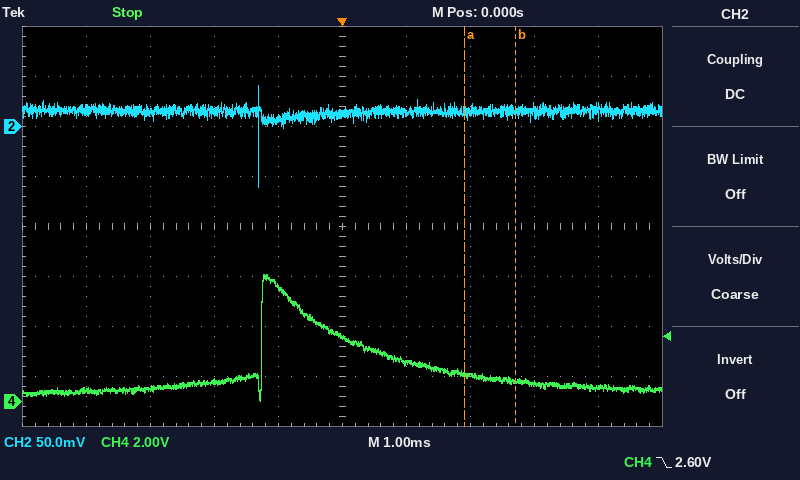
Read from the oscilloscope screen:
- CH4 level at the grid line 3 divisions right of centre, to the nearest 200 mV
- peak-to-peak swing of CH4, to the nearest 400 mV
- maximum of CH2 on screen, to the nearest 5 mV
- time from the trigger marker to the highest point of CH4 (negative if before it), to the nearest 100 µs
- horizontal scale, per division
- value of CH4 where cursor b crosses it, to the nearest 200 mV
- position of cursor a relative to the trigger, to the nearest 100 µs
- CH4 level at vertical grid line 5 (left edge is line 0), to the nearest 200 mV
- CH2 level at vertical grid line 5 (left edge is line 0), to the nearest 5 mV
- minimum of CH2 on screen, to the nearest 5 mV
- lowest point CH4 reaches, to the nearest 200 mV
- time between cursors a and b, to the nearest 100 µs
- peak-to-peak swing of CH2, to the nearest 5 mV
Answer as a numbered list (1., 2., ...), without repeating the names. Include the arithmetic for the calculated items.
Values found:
1. 800 mV
2. 5.2 V
3. 40 mV
4. -1.2 ms
5. 1 ms
6. 800 mV
7. +1.9 ms
8. 2.6 V
9. 15 mV
10. -60 mV
11. 0.0 V
12. 800 µs
13. 40 mV − (-60 mV) = 100 mV
